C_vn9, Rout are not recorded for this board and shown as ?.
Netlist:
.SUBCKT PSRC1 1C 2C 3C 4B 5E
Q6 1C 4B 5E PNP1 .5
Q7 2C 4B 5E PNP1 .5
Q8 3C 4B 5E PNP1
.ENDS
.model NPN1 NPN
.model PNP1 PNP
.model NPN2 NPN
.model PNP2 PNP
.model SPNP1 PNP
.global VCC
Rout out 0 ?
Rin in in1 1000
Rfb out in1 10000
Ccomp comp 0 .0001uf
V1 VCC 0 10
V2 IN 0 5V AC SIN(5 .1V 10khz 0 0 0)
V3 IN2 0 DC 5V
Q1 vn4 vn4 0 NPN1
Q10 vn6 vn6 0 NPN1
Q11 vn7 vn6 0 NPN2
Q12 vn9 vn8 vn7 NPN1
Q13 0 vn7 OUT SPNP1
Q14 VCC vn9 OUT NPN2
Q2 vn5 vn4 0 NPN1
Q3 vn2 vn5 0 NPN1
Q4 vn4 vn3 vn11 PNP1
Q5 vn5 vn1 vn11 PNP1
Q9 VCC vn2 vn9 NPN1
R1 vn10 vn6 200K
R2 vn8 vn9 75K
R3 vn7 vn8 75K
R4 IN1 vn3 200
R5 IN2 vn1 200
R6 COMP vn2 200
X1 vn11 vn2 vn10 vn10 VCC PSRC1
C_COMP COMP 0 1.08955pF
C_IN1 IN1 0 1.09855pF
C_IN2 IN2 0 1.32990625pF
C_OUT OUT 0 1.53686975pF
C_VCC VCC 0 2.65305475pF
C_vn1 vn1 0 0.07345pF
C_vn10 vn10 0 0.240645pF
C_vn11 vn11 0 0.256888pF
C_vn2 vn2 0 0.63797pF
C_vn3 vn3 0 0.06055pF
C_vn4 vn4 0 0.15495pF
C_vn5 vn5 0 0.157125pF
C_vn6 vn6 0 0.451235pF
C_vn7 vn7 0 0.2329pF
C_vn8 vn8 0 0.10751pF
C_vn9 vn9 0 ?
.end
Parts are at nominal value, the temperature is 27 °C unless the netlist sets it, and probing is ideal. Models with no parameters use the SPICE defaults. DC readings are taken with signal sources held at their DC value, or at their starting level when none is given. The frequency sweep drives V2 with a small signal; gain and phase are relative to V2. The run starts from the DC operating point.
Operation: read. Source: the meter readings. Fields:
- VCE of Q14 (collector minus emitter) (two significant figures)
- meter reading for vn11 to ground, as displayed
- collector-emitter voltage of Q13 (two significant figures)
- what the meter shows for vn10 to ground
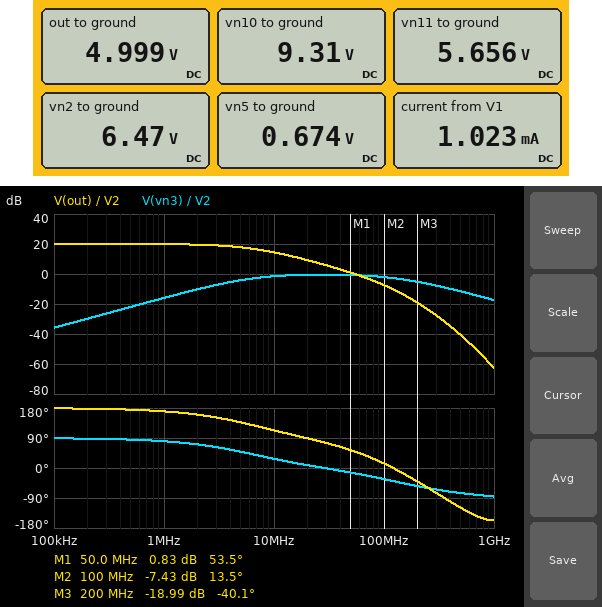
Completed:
5.0 V
5.656 V
-5.0 V
9.31 V
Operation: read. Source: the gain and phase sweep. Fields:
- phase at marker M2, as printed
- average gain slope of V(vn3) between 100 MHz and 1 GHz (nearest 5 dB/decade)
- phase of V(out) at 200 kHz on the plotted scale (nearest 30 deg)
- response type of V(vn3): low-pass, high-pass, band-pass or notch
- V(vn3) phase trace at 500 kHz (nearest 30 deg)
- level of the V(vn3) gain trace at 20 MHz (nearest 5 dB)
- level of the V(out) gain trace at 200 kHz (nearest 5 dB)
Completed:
13.5 deg
-15 dB/decade
180 deg
band-pass
90 deg
0 dB
20 dB
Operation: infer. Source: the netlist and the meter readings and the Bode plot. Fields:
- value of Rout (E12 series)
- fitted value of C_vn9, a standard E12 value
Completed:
5.6 kΩ
1.8 pF
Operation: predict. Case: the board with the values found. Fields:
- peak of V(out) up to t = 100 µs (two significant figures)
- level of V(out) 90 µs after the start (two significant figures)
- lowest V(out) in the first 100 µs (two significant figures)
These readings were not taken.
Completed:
6.0 V
5.6 V
4.0 V
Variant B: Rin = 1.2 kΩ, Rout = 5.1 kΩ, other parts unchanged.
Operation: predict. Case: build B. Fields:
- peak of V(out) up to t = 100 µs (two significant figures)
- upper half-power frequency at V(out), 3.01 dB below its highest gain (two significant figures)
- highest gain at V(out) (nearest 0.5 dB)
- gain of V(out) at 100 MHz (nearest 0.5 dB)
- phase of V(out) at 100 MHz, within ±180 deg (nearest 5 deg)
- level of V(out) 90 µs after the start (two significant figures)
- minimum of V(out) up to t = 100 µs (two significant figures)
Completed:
5.8 V
7.5 MHz
18.5 dB
-8.0 dB
10 deg
5.5 V
4.2 V
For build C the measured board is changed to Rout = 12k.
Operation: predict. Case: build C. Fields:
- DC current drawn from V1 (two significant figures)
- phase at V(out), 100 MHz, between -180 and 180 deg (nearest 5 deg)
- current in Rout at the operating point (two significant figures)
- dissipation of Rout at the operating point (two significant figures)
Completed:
550 µA
10 deg
420 µA
2.1 mW
